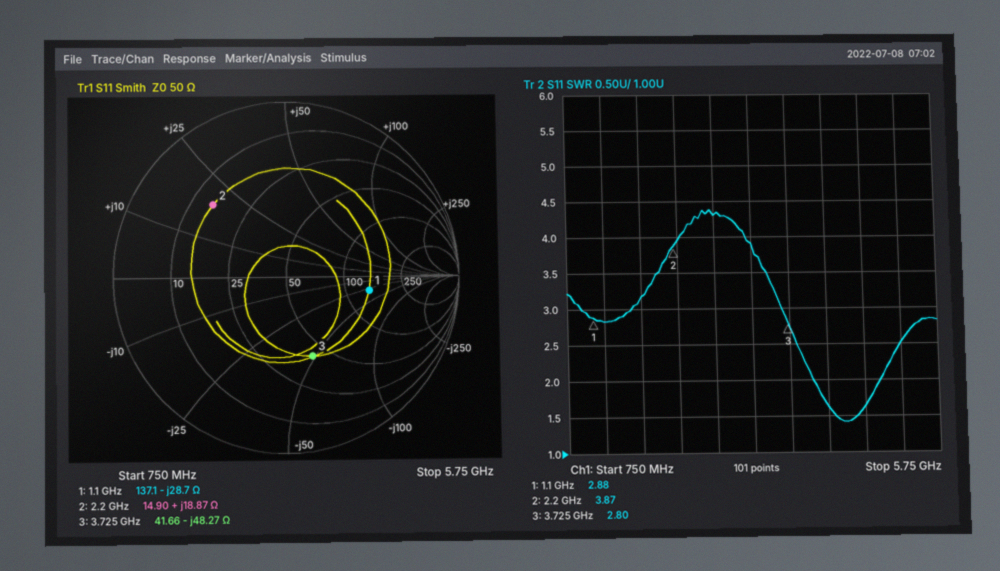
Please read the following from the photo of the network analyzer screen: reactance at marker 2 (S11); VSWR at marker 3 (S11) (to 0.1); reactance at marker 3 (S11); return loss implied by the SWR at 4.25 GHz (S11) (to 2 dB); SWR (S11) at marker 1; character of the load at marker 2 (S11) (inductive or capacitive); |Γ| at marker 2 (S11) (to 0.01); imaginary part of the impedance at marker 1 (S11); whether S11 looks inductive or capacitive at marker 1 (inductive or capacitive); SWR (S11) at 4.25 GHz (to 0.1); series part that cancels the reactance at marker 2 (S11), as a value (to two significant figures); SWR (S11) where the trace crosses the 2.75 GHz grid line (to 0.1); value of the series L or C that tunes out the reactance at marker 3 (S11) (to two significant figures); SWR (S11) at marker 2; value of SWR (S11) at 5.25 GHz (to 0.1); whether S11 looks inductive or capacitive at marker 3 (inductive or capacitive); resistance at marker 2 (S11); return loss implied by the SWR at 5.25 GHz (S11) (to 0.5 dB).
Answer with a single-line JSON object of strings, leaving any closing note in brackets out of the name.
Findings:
{"reactance at marker 2": "+18.87 Ω", "VSWR at marker 3 (S11)": "2.8", "reactance at marker 3": "-48.27 Ω", "return loss implied by the SWR at 4.25 GHz (S11)": "12 dB", "SWR (S11) at marker 1": "2.88", "character of the load at marker 2 (S11)": "inductive", "|Γ| at marker 2 (S11)": "0.59", "imaginary part of the impedance at marker 1": "-28.7 Ω", "whether S11 looks inductive or capacitive at marker 1": "capacitive", "SWR (S11) at 4.25 GHz": "1.6", "series part that cancels the reactance at marker 2 (S11), as a value": "3.8 pF", "SWR (S11) where the trace crosses the 2.75 GHz grid line": "4.3", "value of the series L or C that tunes out the reactance at marker 3 (S11)": "2.1 nH", "SWR (S11) at marker 2": "3.87", "value of SWR (S11) at 5.25 GHz": "2.5", "whether S11 looks inductive or capacitive at marker 3": "capacitive", "resistance at marker 2": "14.90 Ω", "return loss implied by the SWR at 5.25 GHz (S11)": "7.5 dB"}
